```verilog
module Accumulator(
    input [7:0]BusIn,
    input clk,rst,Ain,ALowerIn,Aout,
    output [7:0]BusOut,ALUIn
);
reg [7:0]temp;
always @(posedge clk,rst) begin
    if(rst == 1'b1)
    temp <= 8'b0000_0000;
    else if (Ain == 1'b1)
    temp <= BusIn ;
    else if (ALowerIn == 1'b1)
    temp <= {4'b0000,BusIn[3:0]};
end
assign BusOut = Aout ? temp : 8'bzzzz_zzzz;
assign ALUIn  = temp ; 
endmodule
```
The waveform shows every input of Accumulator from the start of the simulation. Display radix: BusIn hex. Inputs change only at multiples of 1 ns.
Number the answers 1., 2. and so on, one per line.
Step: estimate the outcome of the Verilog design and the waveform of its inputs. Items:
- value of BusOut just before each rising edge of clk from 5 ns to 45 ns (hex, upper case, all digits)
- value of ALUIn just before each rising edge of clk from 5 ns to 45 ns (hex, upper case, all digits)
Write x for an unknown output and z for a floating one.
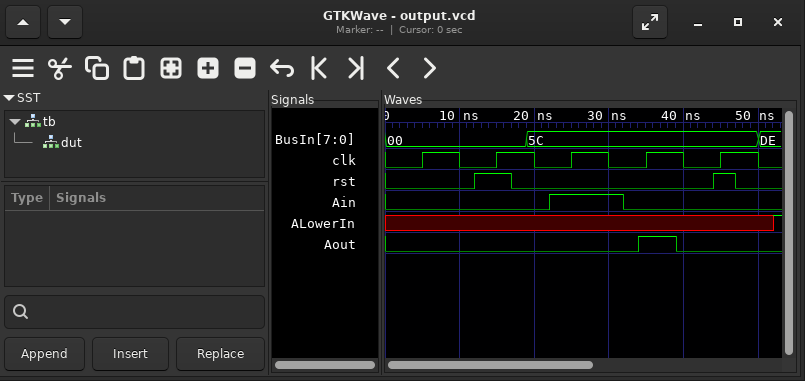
1. z, z, z, 5C, z
2. x, 00, 00, 5C, 00
